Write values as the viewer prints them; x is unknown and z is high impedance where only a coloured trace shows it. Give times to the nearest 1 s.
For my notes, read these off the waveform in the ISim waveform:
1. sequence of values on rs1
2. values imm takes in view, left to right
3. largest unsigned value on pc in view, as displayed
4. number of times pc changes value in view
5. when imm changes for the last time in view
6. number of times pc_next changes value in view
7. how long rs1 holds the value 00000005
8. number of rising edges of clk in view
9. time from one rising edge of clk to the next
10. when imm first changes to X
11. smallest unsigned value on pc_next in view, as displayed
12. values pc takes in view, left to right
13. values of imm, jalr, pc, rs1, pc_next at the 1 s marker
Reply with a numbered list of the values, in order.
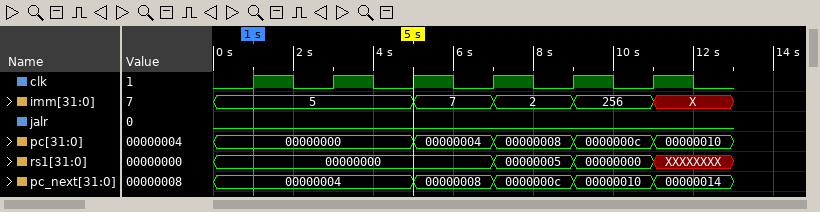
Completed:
1. 00000000, 00000005, 00000000, XXXXXXXX
2. 5, 7, 2, 256, X
3. 00000010
4. 4
5. 11 s
6. 4
7. 2 s
8. 6
9. 2 s
10. 11 s
11. 00000004
12. 00000000, 00000004, 00000008, 0000000c, 00000010
13. imm=5, jalr=0, pc=00000000, rs1=00000000, pc_next=00000004
